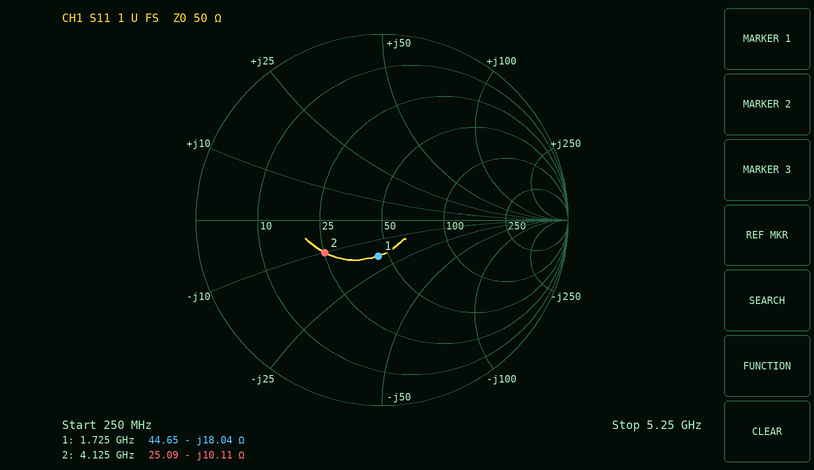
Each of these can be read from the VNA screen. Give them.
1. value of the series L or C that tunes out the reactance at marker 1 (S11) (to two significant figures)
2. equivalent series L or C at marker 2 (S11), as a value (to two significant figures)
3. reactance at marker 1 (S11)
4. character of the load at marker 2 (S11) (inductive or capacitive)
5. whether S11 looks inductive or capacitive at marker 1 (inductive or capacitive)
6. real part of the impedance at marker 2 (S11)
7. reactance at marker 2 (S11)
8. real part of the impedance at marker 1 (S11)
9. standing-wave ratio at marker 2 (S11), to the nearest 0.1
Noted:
1.7 nH
3.8 pF
-18.04 Ω
capacitive
capacitive
25.09 Ω
-10.11 Ω
44.65 Ω
2.1
